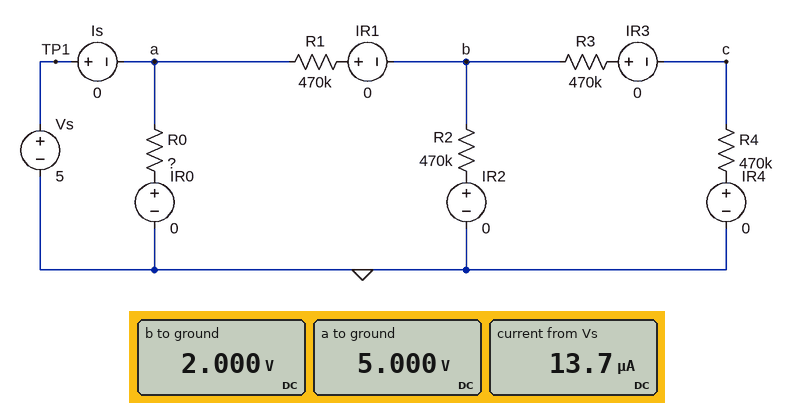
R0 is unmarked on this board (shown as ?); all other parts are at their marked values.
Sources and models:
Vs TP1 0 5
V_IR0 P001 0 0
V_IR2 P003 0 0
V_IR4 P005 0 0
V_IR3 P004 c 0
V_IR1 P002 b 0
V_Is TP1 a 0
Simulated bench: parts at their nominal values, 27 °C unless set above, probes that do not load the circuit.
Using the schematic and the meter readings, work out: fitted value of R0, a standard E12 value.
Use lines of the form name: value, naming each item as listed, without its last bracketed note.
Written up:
fitted value of R0, a standard E12 value: 680 kΩ
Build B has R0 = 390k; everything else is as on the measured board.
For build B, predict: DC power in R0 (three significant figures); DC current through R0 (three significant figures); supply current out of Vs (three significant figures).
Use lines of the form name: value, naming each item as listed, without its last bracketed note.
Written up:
DC power in R0: 64.1 µW
DC current through R0: 12.8 µA
supply current out of Vs: 19.2 µA
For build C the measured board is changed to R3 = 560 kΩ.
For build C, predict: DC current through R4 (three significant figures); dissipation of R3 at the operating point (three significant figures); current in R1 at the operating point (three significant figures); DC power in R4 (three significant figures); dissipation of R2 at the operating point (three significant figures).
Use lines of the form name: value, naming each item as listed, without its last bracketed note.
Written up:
DC current through R4: 1.98 µA
dissipation of R3 at the operating point: 2.19 µW
current in R1 at the operating point: 6.31 µA
DC power in R4: 1.84 µW
dissipation of R2 at the operating point: 8.82 µW
